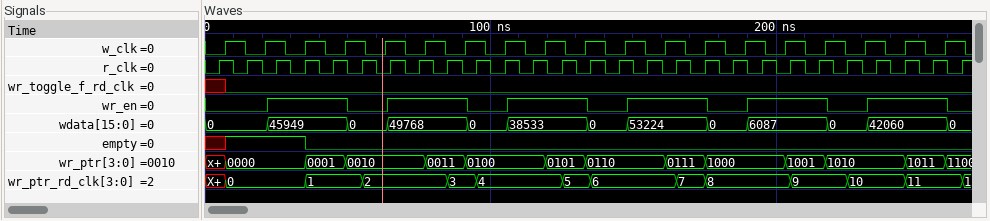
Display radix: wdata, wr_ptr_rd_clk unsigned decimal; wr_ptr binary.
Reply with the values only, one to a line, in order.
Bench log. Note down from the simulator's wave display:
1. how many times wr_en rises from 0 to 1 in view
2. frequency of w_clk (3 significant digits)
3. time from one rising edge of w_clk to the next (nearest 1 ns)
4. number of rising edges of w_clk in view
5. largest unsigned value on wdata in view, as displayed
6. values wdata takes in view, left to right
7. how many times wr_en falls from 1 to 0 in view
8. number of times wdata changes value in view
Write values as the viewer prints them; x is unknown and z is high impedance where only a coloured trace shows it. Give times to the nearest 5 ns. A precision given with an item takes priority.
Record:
6
71.4 MHz
14 ns
19
53224
0, 45949, 0, 49768, 0, 38533, 0, 53224, 0, 6087, 0, 42060, 0
6
12
